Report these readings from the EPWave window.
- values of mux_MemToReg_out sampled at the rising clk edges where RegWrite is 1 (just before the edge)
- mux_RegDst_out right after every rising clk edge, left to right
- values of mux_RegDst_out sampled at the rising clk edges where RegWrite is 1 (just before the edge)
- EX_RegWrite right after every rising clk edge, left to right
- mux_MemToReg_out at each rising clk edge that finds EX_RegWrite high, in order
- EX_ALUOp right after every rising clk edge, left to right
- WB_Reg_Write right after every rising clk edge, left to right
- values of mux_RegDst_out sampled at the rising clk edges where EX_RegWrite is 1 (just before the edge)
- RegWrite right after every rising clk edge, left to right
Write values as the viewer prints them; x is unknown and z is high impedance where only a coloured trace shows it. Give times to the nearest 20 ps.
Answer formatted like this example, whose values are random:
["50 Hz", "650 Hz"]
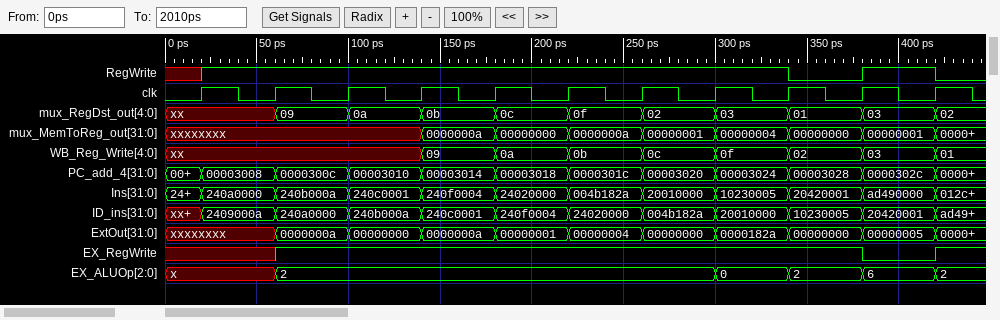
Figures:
["xxxxxxxx, xxxxxxxx, xxxxxxxx, 0000000a, 00000000, 0000000a, 00000001, 00000004, 00000001", "xx, 09, 0a, 0b, 0c, 0f, 02, 03, 01, 03, 02", "xx, 09, 0a, 0b, 0c, 0f, 02, 03, 03", "x 1 1 1 1 1 1 1 1 0 1", "xxxxxxxx, xxxxxxxx, 0000000a, 00000000, 0000000a, 00000001, 00000004, 00000000", "x, 2, 2, 2, 2, 2, 2, 0, 2, 6, 2", "xx, xx, xx, 09, 0a, 0b, 0c, 0f, 02, 03, 01", "09, 0a, 0b, 0c, 0f, 02, 03, 01", "1 1 1 1 1 1 1 1 0 1 0"]
